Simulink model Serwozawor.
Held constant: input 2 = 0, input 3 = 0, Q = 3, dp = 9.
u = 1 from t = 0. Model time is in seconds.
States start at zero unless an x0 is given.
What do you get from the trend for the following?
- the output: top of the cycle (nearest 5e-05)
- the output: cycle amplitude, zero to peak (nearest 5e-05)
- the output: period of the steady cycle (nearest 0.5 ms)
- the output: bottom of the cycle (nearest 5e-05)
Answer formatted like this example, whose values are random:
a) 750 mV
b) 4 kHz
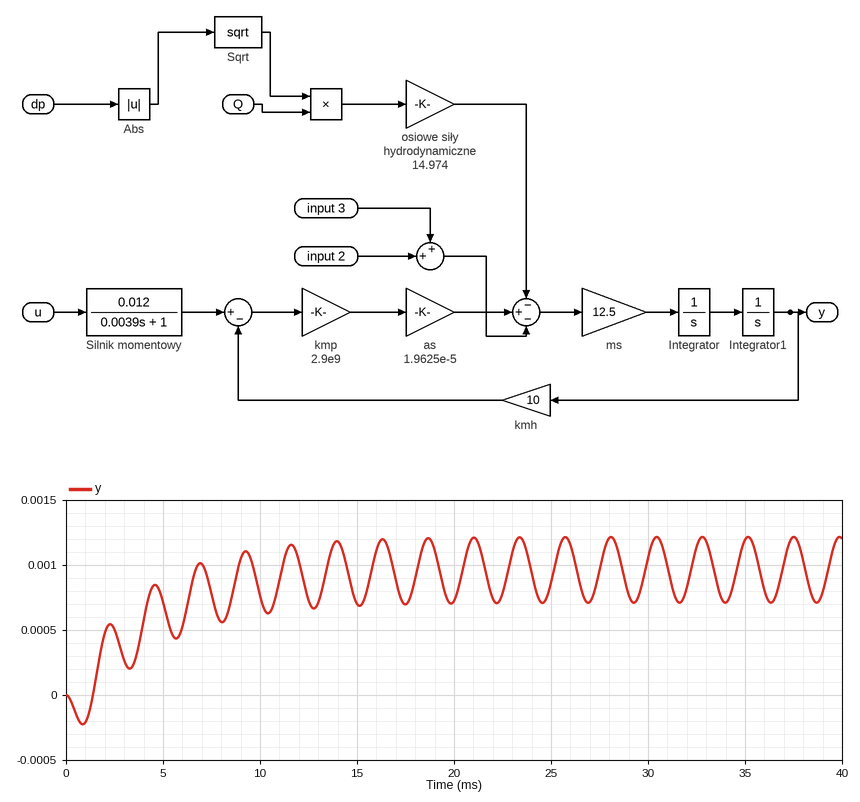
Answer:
a) 0.00120
b) 0.00025
c) 2.5 ms
d) 0.00070
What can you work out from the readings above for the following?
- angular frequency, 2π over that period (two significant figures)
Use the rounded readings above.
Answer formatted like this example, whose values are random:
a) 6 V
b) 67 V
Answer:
a) 2.5 rad/ms
